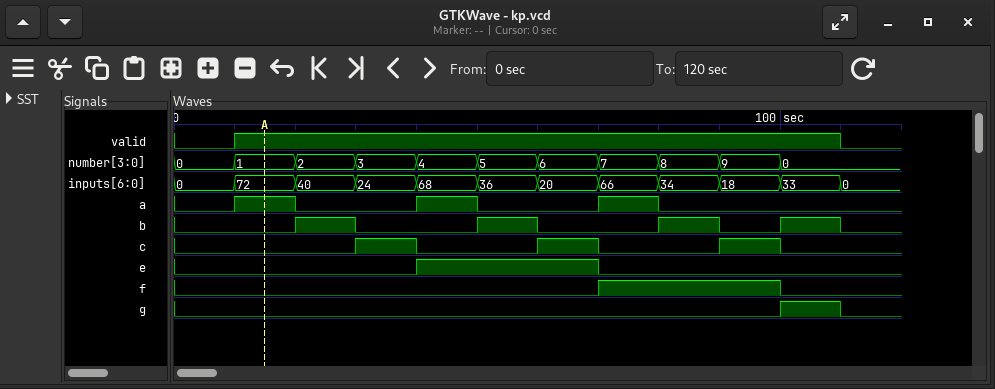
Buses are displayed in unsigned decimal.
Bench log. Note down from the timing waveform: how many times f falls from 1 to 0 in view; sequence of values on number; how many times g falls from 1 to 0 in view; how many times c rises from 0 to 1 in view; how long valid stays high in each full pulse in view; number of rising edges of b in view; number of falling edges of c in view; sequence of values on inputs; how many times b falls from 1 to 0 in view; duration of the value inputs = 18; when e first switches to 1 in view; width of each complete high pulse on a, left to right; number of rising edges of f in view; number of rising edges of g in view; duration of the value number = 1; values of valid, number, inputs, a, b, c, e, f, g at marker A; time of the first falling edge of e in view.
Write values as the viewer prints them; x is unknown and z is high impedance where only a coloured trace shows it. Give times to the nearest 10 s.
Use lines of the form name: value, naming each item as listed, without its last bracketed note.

how many times f falls from 1 to 0 in view: 1
sequence of values on number: 0, 1, 2, 3, 4, 5, 6, 7, 8, 9, 0
how many times g falls from 1 to 0 in view: 1
how many times c rises from 0 to 1 in view: 3
how long valid stays high in each full pulse in view: 100 s
number of rising edges of b in view: 4
number of falling edges of c in view: 3
sequence of values on inputs: 0, 72, 40, 24, 68, 36, 20, 66, 34, 18, 33, 0
how many times b falls from 1 to 0 in view: 4
duration of the value inputs = 18: 10 s
when e first switches to 1 in view: 40 s
width of each complete high pulse on a, left to right: 10 s, 10 s, 10 s
number of rising edges of f in view: 1
number of rising edges of g in view: 1
duration of the value number = 1: 10 s
values of valid, number, inputs, a, b, c, e, f, g at marker A: valid=1, number=1, inputs=72, a=1, b=0, c=0, e=0, f=0, g=0
time of the first falling edge of e in view: 70 s
